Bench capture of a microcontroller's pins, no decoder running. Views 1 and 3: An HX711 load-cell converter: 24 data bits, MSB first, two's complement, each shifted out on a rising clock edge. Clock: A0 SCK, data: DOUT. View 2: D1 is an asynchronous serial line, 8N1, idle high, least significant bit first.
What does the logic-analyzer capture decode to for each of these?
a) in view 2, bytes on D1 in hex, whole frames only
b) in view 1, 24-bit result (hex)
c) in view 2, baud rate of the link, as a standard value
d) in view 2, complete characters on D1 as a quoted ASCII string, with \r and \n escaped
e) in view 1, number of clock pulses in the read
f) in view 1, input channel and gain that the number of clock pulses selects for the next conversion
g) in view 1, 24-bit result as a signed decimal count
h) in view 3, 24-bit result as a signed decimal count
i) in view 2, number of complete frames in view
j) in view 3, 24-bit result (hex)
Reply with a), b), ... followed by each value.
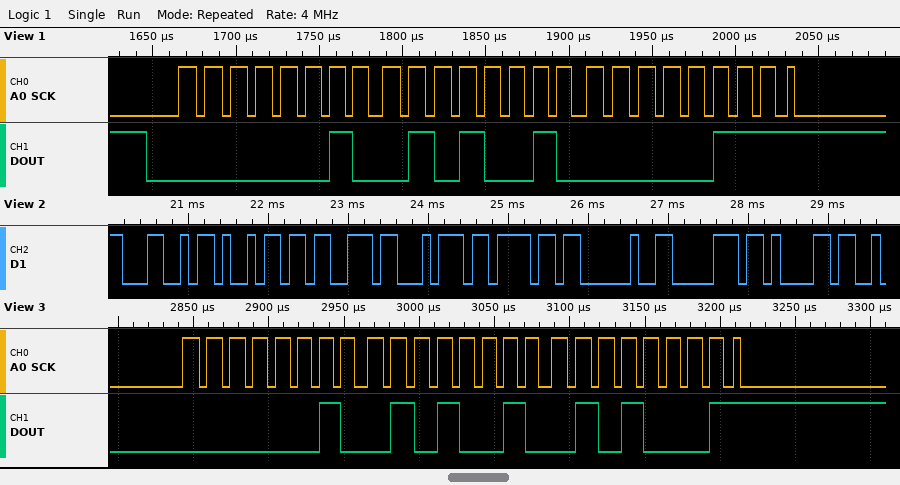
a) 4C 69 73 74 6F 20 70 61
b) 0x025207
c) 9600 baud
d) "Listo pa"
e) 25
f) channel A, gain 128
g) 152071
h) 152145
i) 8
j) 0x025251
